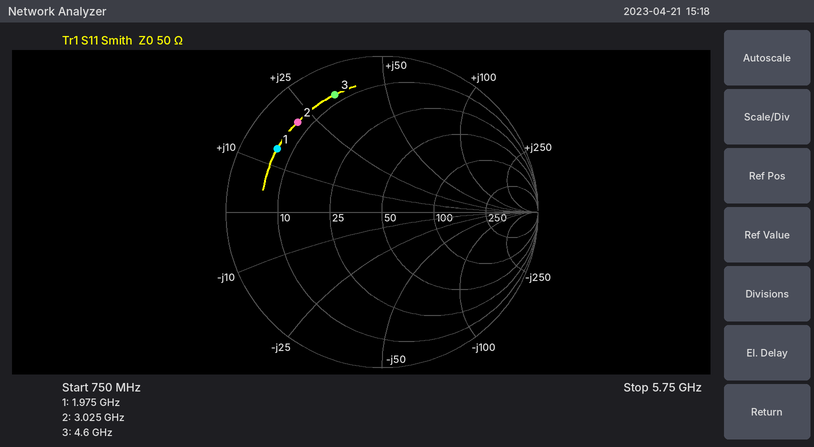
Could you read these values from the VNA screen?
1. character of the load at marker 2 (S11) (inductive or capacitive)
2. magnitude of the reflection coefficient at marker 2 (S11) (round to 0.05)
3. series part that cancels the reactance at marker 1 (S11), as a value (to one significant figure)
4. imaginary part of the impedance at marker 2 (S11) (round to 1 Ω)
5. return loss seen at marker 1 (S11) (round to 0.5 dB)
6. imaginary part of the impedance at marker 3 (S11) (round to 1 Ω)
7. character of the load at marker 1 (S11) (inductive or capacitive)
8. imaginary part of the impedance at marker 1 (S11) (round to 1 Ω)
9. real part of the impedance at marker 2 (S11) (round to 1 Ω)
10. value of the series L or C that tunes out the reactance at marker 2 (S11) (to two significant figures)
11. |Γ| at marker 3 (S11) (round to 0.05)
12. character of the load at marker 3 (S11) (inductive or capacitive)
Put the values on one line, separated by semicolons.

inductive; 0.80; 6 pF; +21 Ω; 2.0 dB; +33 Ω; inductive; +14 Ω; 7 Ω; 2.5 pF; 0.80; inductive
